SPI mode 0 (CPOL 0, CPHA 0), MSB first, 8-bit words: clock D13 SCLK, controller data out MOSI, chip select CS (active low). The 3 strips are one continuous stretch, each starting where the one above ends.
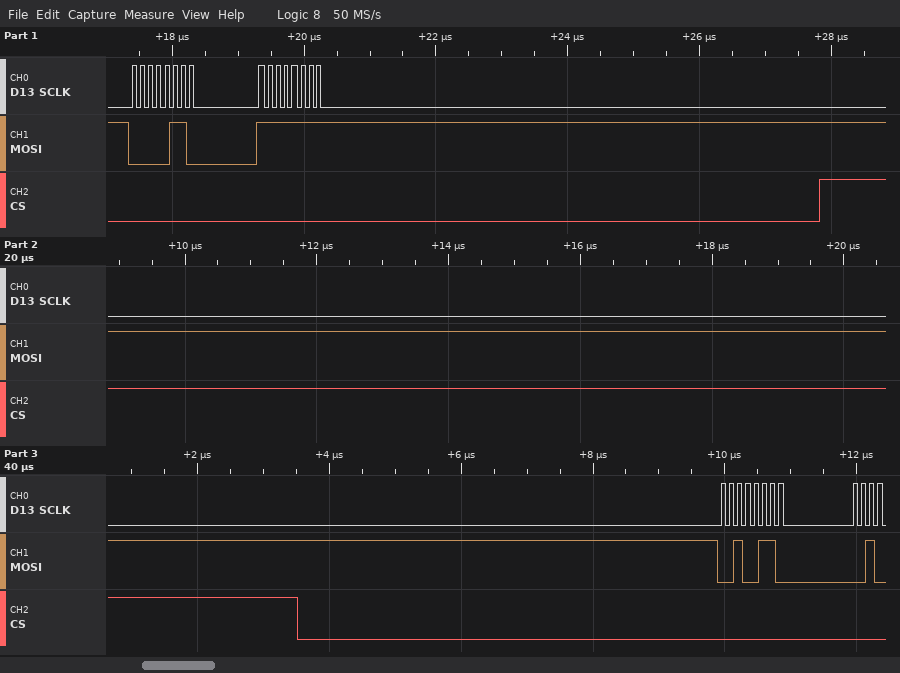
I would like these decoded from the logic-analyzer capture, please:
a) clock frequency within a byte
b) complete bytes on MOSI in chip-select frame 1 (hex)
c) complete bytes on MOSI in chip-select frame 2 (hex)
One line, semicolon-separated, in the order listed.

8 MHz; 06 FF; 26
